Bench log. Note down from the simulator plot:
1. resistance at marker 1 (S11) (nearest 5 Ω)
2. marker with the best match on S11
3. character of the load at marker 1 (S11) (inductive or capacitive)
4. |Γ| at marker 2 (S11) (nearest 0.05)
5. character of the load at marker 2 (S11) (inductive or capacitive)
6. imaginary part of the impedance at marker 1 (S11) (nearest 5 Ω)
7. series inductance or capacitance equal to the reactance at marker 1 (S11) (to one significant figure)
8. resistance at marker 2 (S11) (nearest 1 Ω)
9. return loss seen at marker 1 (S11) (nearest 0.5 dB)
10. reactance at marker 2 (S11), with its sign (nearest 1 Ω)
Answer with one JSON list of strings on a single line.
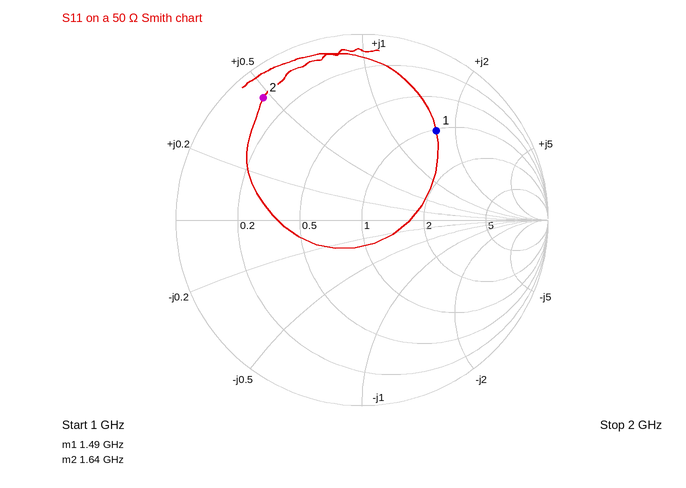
["50 Ω", "marker 1", "inductive", "0.85", "inductive", "+80 Ω", "9 nH", "5 Ω", "4.0 dB", "+24 Ω"]
